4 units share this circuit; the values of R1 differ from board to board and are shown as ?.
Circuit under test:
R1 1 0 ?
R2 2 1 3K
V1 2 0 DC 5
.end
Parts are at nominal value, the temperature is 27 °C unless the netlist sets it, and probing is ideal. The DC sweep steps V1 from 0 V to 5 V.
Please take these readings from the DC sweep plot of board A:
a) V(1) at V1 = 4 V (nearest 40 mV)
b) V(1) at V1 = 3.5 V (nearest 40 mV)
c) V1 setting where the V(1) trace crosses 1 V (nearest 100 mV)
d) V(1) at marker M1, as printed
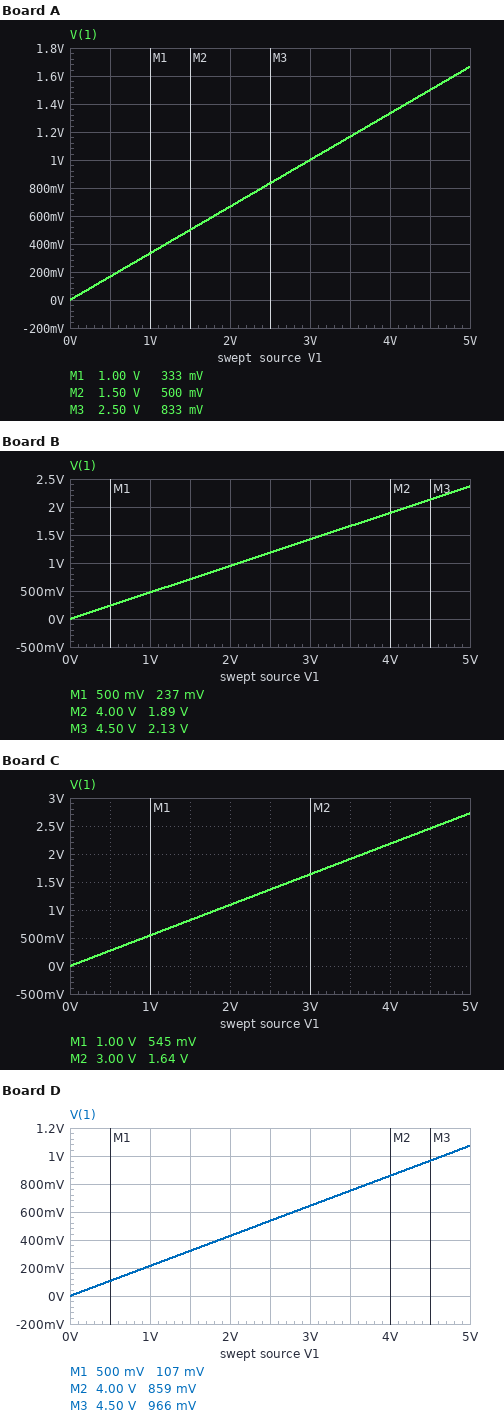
1.32 V
1.16 V
3.0 V
333 mV
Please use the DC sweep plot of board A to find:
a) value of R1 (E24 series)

1.5 kΩ
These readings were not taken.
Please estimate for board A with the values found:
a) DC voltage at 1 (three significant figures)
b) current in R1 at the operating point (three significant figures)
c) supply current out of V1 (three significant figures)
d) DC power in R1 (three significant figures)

1.67 V
1.11 mA
1.11 mA
1.85 mW
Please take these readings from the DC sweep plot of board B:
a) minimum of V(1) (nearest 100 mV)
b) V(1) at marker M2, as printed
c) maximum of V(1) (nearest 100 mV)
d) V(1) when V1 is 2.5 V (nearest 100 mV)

0 V
1.89 V
2.4 V
1.2 V
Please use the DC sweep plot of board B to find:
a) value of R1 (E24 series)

2.7 kΩ
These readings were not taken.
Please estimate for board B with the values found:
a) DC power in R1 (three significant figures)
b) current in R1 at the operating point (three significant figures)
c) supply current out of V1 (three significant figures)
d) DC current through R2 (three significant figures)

2.08 mW
877 µA
877 µA
877 µA
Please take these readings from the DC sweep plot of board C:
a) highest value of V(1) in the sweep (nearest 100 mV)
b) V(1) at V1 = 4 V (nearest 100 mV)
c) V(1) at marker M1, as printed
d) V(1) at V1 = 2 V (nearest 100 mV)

2.7 V
2.2 V
545 mV
1.1 V
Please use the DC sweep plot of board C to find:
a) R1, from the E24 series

3.6 kΩ
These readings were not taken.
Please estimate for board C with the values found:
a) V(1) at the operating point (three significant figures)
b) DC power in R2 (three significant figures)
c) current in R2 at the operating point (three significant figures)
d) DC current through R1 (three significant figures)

2.73 V
1.72 mW
758 µA
758 µA
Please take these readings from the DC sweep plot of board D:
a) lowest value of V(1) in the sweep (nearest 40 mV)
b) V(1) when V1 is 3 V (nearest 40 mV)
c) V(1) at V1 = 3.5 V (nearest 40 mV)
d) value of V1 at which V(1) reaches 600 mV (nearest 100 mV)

0 V
640 mV
760 mV
2.8 V
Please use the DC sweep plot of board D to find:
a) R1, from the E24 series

820 Ω
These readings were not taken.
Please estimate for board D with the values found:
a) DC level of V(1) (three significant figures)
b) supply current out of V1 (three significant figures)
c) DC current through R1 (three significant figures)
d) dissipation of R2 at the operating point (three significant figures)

1.07 V
1.31 mA
1.31 mA
5.14 mW
